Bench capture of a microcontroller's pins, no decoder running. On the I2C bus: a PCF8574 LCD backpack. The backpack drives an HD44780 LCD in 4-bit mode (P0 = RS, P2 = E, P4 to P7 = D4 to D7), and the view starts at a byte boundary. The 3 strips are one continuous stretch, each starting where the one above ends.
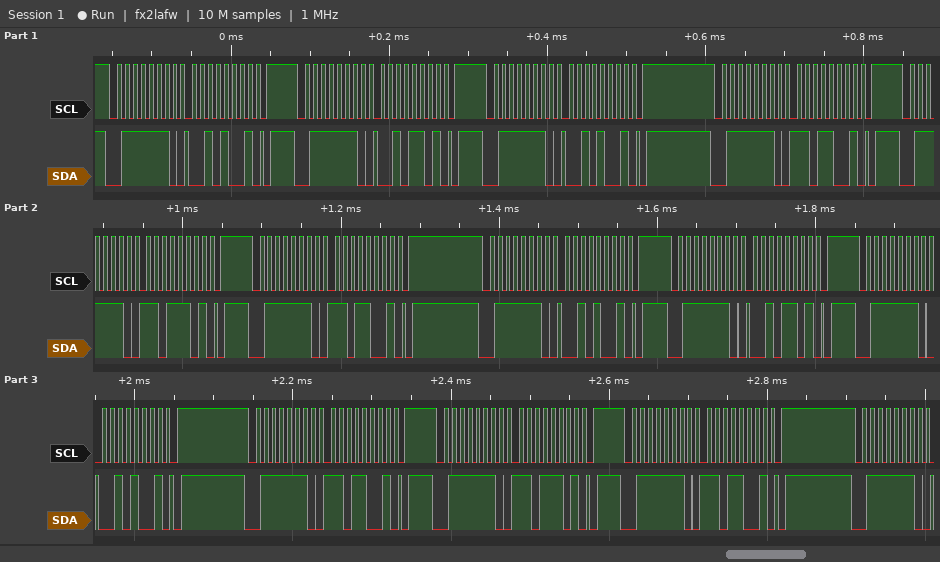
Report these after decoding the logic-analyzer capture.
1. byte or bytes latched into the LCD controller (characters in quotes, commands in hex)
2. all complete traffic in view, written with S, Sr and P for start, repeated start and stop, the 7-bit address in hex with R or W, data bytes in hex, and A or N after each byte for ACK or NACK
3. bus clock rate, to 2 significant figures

'-' '-'
S 3FW A 29 A P S 3FW A 2D A P S 3FW A 29 A P S 3FW A D9 A P S 3FW A DD A P S 3FW A D9 A P S 3FW A 29 A P S 3FW A 2D A P S 3FW A 29 A P S 3FW A D9 A P S 3FW A DD A P S 3FW A D9 A P S 3FW A
100 kHz
